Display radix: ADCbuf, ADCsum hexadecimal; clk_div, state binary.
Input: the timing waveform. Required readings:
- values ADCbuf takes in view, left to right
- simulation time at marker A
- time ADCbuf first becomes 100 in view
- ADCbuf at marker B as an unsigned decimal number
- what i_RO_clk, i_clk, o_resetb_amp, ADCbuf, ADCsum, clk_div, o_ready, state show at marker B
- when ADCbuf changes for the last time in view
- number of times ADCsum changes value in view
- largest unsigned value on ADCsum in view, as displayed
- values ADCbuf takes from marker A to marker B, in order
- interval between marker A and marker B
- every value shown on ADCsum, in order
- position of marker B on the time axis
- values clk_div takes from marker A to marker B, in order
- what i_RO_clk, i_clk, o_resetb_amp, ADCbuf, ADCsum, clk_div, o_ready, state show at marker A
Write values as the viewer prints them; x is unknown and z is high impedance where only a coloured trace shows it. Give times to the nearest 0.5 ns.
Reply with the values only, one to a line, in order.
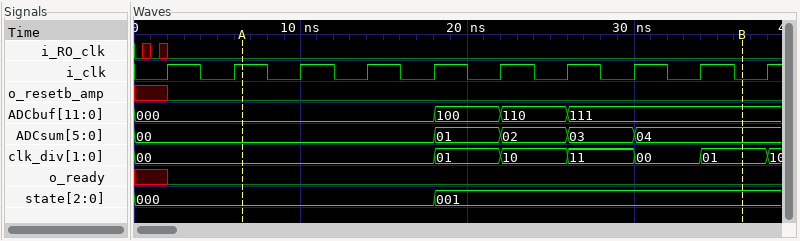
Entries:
000, 100, 110, 111
6.5 ns
18 ns
273
i_RO_clk=0, i_clk=0, o_resetb_amp=0, ADCbuf=111, ADCsum=04, clk_div=01, o_ready=0, state=001
26 ns
4
04
000, 100, 110, 111
30 ns
00, 01, 02, 03, 04
36.5 ns
00, 01, 10, 11, 00, 01
i_RO_clk=0, i_clk=1, o_resetb_amp=0, ADCbuf=000, ADCsum=00, clk_div=00, o_ready=0, state=000
